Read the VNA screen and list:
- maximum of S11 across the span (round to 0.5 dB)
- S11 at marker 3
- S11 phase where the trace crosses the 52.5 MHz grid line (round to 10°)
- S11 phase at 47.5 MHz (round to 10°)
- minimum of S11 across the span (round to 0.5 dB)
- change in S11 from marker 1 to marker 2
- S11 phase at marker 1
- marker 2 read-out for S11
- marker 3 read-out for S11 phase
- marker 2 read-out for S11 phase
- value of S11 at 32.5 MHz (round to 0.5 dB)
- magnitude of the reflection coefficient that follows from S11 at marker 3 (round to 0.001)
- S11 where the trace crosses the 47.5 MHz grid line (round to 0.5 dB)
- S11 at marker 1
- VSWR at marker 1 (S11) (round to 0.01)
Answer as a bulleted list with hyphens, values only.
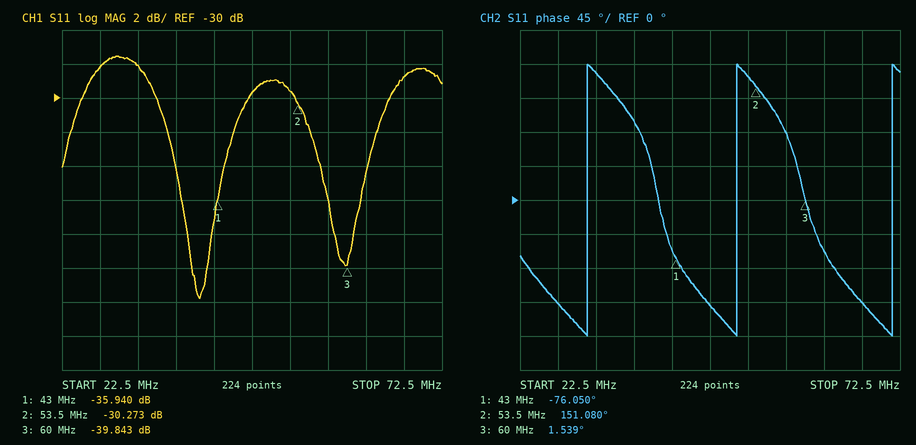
- -27.5 dB
- -39.843 dB
- 160°
- -140°
- -42.0 dB
- 5.667 dB
- -76.050°
- -30.273 dB
- 1.539°
- 151.080°
- -28.0 dB
- 0.010
- -29.5 dB
- -35.940 dB
- 1.03
